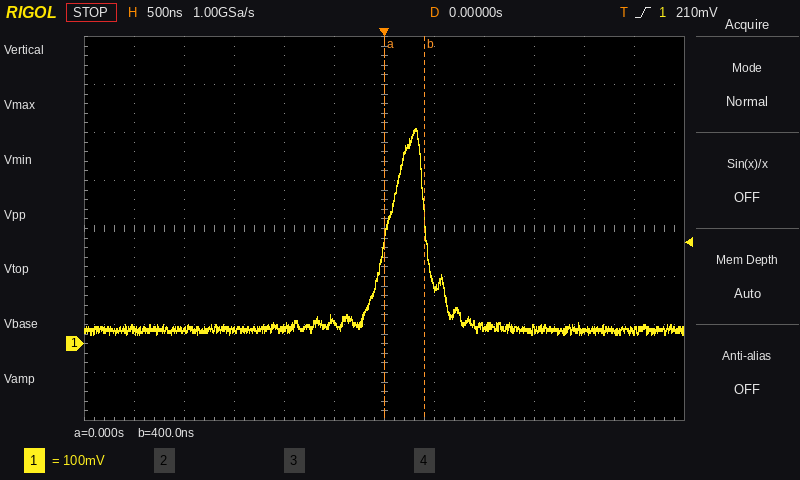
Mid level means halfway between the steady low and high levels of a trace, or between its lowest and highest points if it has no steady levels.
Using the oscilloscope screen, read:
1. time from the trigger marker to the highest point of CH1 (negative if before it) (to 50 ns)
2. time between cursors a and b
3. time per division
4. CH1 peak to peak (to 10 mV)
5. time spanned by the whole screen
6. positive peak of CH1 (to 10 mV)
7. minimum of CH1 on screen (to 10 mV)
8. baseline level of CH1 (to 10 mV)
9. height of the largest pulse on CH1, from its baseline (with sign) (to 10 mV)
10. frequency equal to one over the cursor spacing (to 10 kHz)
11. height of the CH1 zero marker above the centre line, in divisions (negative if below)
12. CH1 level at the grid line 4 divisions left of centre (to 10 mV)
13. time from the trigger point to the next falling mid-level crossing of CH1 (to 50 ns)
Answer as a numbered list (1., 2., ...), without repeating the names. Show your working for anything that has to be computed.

1. +300 ns
2. 400 ns − (0 s) = 400 ns
3. 500 ns
4. 450 mV − (20 mV) = 430 mV
5. 6 µs
6. 450 mV
7. 20 mV
8. 30 mV
9. 450 mV − (30 mV) = +420 mV
10. 1 / 400 ns ≈ 2.50 MHz
11. -2.4 div
12. 30 mV
13. 400 ns
